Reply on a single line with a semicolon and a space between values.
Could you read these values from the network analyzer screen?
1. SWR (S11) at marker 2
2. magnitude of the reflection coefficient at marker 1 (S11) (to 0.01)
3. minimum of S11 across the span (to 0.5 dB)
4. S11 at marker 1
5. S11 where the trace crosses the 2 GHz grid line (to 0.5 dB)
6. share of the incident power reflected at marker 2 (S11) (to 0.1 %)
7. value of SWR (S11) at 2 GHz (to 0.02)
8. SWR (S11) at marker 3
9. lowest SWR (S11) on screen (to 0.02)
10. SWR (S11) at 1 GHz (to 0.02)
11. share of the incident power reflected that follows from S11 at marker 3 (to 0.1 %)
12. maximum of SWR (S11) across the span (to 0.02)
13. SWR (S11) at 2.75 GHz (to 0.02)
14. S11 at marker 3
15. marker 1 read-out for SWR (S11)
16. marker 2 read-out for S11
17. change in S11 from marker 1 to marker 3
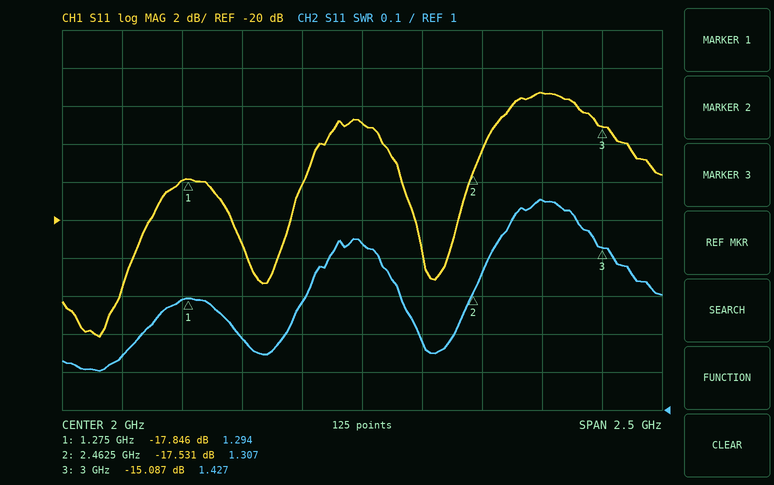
1.307; 0.13; -26.0 dB; -17.846 dB; -15.0 dB; 1.8 %; 1.44; 1.427; 1.10; 1.14; 3.1 %; 1.56; 1.56; -15.087 dB; 1.294; -17.531 dB; 2.759 dB
